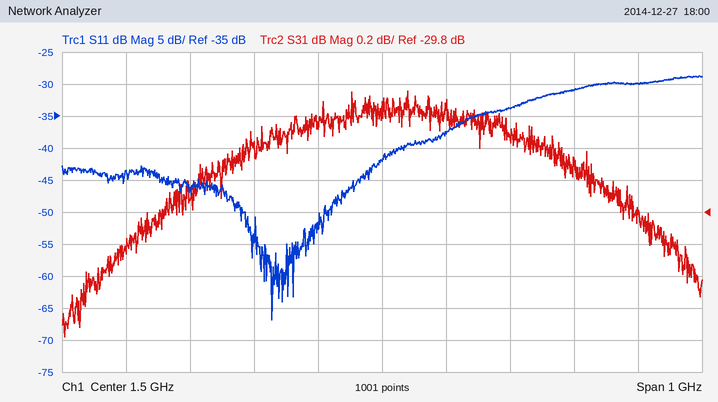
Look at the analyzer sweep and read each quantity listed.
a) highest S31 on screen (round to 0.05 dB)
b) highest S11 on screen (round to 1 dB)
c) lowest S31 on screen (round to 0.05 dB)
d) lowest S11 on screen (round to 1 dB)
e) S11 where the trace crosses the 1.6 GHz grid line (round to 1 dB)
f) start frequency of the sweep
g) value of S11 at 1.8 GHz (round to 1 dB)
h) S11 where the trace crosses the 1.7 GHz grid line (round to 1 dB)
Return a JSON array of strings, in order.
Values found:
["-29.05 dB", "-29 dB", "-30.60 dB", "-67 dB", "-38 dB", "1 GHz", "-31 dB", "-34 dB"]
